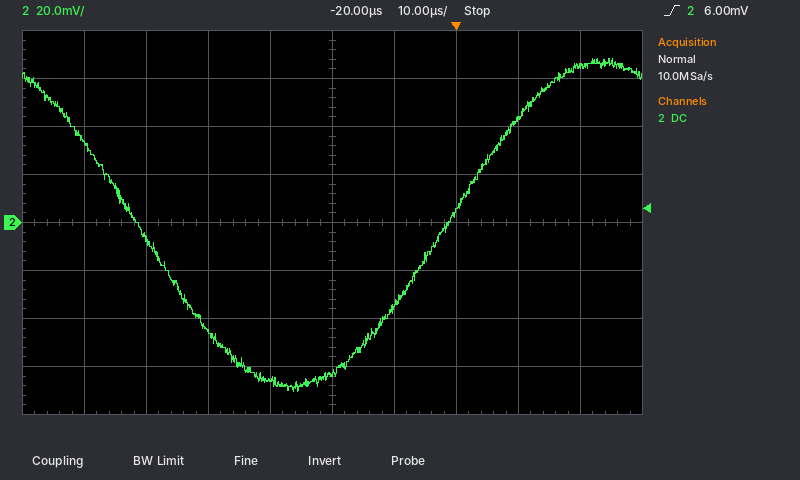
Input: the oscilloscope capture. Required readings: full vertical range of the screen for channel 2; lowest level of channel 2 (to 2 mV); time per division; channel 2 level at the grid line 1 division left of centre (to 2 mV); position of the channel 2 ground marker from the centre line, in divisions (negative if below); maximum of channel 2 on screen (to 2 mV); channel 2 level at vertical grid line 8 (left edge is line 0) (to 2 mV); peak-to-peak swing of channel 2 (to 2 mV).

160 mV
-70 mV
10 µs
-66 mV
0.0 div
68 mV
42 mV
138 mV
